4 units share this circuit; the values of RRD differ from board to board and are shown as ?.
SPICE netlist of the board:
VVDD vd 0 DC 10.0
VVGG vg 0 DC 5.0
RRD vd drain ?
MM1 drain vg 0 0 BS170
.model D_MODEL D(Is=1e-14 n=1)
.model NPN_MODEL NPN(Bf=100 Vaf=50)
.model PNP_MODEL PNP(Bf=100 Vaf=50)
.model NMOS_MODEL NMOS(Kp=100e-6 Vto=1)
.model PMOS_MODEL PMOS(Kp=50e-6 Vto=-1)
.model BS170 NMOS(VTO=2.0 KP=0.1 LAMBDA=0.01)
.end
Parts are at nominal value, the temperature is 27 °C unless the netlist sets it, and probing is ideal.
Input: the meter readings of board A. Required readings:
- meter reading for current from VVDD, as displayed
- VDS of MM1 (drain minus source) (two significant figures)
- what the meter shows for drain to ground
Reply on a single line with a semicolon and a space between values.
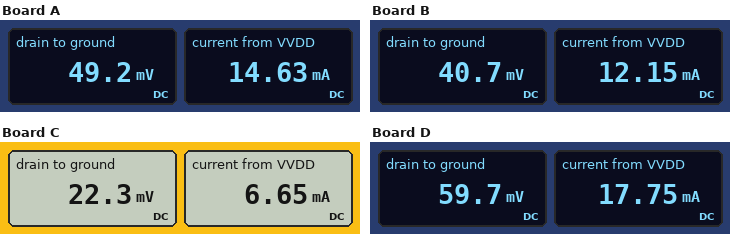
14.63 mA; 49 mV; 49.2 mV
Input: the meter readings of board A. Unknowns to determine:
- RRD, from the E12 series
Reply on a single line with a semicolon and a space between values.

680 Ω
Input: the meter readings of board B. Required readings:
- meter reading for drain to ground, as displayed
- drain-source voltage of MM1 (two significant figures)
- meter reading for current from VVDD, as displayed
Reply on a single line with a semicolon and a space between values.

40.7 mV; 41 mV; 12.15 mA
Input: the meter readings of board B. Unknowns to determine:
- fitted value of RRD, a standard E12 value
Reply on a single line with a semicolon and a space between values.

820 Ω
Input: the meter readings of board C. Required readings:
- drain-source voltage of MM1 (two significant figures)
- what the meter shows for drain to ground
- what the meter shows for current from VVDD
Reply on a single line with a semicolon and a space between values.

22 mV; 22.3 mV; 6.65 mA
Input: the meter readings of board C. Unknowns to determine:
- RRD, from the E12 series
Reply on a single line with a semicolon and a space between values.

1.5 kΩ
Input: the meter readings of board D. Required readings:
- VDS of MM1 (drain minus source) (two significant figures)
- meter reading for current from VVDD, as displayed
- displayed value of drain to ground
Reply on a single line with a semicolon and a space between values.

60 mV; 17.75 mA; 59.7 mV
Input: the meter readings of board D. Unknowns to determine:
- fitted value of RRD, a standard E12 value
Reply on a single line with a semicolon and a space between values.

560 Ω
